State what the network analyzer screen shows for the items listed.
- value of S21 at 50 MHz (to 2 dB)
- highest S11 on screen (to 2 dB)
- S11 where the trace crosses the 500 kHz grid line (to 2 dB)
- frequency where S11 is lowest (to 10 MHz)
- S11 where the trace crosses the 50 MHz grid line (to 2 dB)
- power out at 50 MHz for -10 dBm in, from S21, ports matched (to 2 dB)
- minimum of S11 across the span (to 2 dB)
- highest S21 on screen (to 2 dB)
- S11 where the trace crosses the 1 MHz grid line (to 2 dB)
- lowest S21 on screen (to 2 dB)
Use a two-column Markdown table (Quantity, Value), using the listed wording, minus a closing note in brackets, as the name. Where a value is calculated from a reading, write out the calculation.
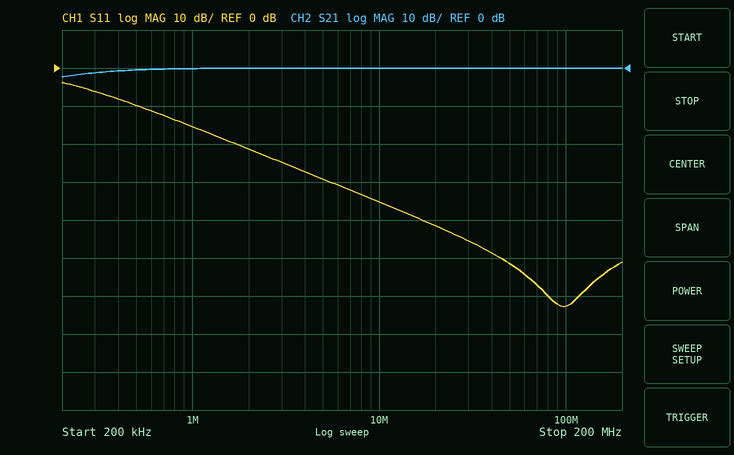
| Quantity | Value |
|---|---|
| value of S21 at 50 MHz | 0 dB |
| highest S11 on screen | -4 dB |
| S11 where the trace crosses the 500 kHz grid line | -10 dB |
| frequency where S11 is lowest | 100 MHz |
| S11 where the trace crosses the 50 MHz grid line | -52 dB |
| power out at 50 MHz for -10 dBm in, from S21, ports matched | -10 dBm + (0 dB) = -10 dBm |
| minimum of S11 across the span | -62 dB |
| highest S21 on screen | 0 dB |
| S11 where the trace crosses the 1 MHz grid line | -16 dB |
| lowest S21 on screen | -2 dB |
